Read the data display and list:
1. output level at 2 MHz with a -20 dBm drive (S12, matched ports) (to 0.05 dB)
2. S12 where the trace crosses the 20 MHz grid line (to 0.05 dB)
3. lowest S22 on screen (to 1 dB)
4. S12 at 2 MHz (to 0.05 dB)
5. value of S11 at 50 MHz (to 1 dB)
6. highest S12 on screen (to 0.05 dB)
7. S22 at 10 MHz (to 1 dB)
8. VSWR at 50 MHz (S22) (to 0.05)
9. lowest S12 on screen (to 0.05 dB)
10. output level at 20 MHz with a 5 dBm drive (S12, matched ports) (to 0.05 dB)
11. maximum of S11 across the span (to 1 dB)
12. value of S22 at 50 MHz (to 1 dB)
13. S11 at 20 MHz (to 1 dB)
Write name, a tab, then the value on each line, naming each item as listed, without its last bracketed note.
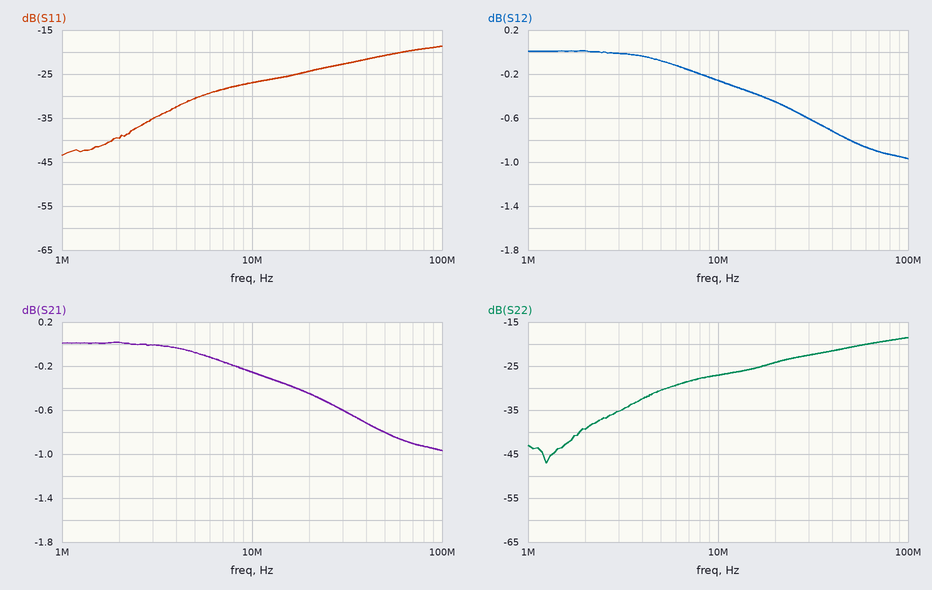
output level at 2 MHz with a -20 dBm drive (S12, matched ports)	-20.00 dBm
S12 where the trace crosses the 20 MHz grid line	-0.45 dB
lowest S22 on screen	-47 dB
S12 at 2 MHz	0.00 dB
value of S11 at 50 MHz	-21 dB
highest S12 on screen	0.00 dB
S22 at 10 MHz	-27 dB
VSWR at 50 MHz (S22)	1.20
lowest S12 on screen	-0.95 dB
output level at 20 MHz with a 5 dBm drive (S12, matched ports)	4.55 dBm
maximum of S11 across the span	-19 dB
value of S22 at 50 MHz	-21 dB
S11 at 20 MHz	-24 dB
